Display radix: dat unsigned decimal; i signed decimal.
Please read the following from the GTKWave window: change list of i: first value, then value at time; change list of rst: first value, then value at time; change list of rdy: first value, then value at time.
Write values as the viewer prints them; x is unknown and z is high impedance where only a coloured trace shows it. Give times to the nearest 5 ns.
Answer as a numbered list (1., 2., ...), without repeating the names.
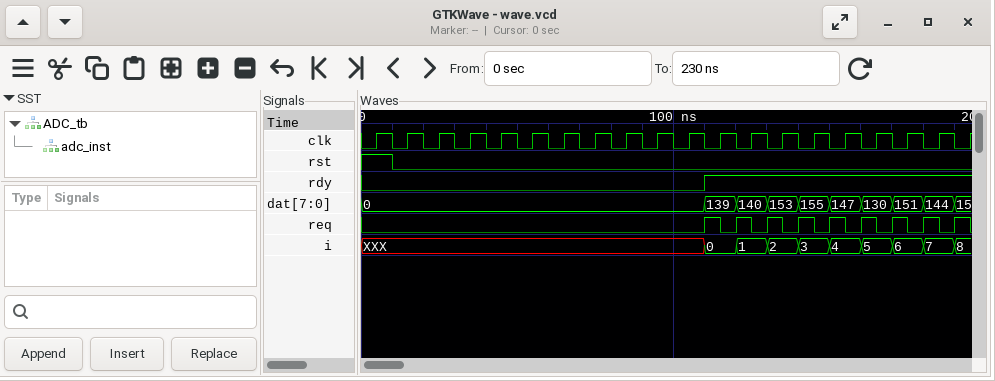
1. XXX, 0 at 110 ns, 1 at 120 ns, 2 at 130 ns, 3 at 140 ns, 4 at 150 ns, 5 at 160 ns, 6 at 170 ns, 7 at 180 ns, 8 at 190 ns
2. 1, 0 at 10 ns
3. 0, 1 at 110 ns
